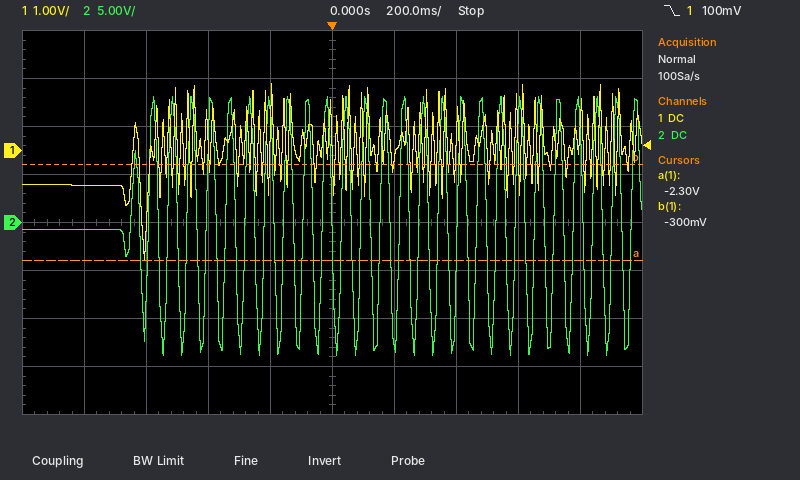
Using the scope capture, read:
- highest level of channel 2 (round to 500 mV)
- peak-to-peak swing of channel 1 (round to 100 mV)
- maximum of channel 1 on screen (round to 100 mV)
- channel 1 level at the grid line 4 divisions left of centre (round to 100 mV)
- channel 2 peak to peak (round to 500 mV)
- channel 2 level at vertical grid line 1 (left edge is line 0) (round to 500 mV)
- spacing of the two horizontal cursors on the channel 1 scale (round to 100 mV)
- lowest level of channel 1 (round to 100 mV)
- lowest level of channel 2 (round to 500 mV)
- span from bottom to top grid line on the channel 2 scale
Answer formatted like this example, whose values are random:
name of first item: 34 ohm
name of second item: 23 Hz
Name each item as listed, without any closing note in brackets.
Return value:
highest level of channel 2: 13.0 V
peak-to-peak swing of channel 1: 3.7 V
maximum of channel 1 on screen: 1.4 V
channel 1 level at the grid line 4 divisions left of centre: -700 mV
channel 2 peak to peak: 27.0 V
channel 2 level at vertical grid line 1 (left edge is line 0): -500 mV
spacing of the two horizontal cursors on the channel 1 scale: 2.0 V
lowest level of channel 1: -2.3 V
lowest level of channel 2: -14.0 V
span from bottom to top grid line on the channel 2 scale: 40 V
